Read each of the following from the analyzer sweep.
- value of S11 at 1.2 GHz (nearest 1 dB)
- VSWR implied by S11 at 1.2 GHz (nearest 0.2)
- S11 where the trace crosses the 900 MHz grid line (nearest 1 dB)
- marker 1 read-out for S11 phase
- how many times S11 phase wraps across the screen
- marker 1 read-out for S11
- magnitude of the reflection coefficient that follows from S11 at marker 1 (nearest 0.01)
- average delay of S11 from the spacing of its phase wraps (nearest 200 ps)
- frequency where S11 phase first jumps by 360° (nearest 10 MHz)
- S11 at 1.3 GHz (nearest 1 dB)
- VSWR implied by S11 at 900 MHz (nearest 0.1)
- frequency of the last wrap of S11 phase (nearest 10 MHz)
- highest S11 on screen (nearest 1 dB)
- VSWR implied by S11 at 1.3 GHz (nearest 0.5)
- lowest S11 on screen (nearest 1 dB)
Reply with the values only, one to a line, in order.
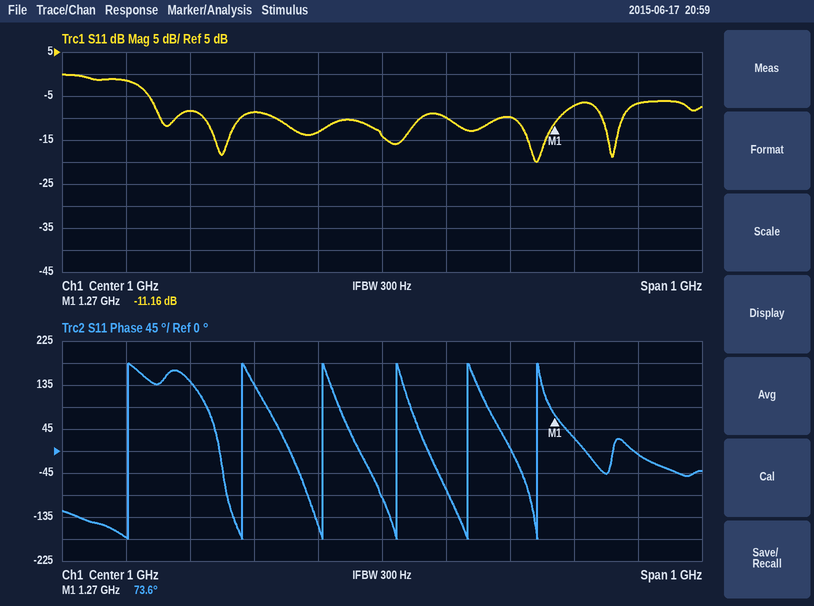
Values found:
-10 dB
2.0
-13 dB
73.6°
6
-11.16 dB
0.28
7.8 ns
600 MHz
-7 dB
1.6
1.24 GHz
0 dB
2.5
-20 dB
